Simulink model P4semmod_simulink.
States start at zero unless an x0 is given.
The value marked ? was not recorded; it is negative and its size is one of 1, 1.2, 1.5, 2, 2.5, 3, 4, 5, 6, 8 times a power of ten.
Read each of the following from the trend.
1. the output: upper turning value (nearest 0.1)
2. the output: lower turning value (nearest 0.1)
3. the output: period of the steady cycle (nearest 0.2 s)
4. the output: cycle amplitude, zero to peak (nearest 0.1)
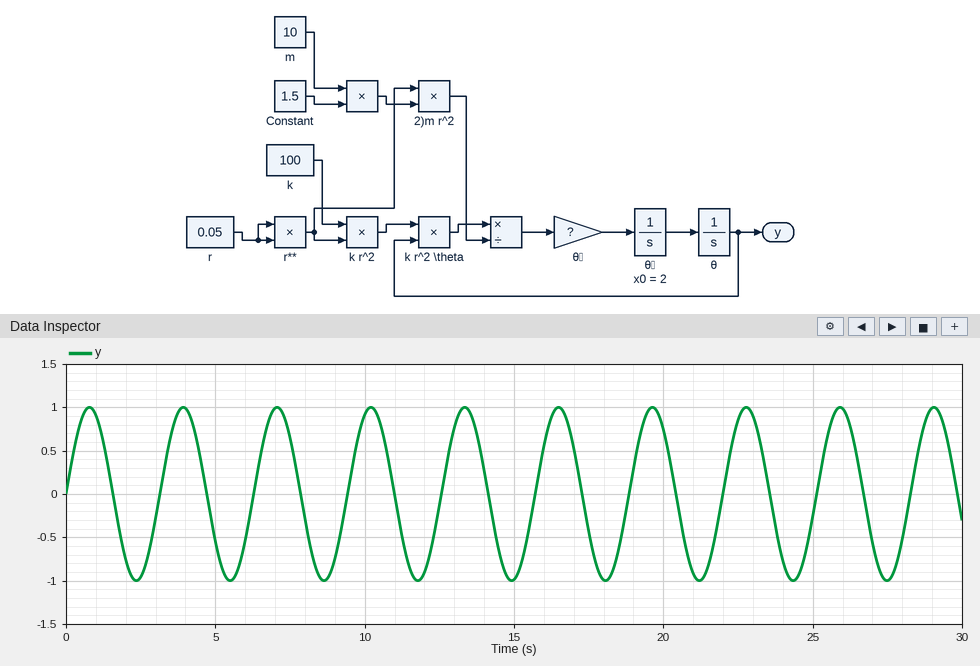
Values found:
1.0
-1.0
3.2 s
1.0
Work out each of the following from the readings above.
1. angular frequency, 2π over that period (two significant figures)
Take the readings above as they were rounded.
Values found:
2.0 rad/s
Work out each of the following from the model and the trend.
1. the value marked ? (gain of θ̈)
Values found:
-0.6
